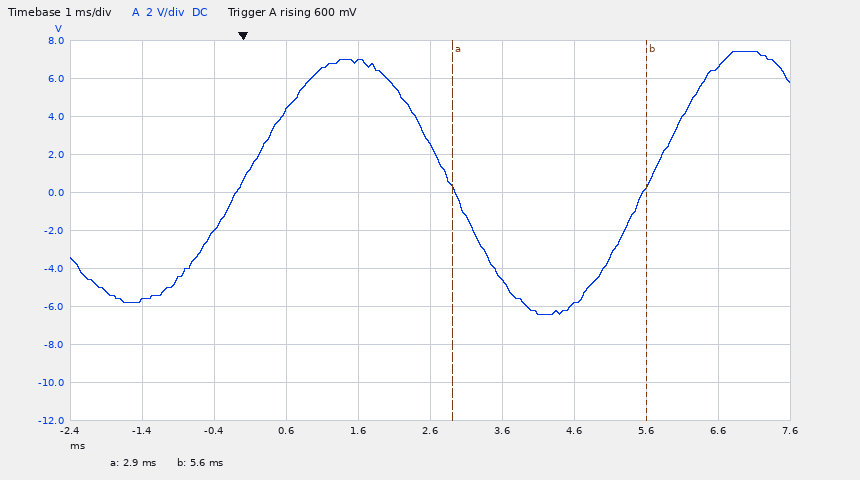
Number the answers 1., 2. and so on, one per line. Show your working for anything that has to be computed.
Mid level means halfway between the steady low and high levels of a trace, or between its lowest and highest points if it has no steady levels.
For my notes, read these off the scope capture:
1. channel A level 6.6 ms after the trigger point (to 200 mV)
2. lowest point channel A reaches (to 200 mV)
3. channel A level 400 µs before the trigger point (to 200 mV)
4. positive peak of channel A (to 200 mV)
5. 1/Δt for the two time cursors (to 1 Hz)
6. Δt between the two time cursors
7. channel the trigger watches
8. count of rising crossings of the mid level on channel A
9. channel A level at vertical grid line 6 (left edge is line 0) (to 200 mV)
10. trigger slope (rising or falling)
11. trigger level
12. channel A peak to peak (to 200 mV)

1. 6.6 V
2. -6.4 V
3. -2.0 V
4. 7.4 V
5. 1 / 2.7 ms ≈ 370 Hz
6. 5.6 ms − (2.9 ms) = 2.7 ms
7. channel A
8. 2
9. -4.6 V
10. rising
11. 600 mV
12. 7.4 V − (-6.4 V) = 13.8 V
